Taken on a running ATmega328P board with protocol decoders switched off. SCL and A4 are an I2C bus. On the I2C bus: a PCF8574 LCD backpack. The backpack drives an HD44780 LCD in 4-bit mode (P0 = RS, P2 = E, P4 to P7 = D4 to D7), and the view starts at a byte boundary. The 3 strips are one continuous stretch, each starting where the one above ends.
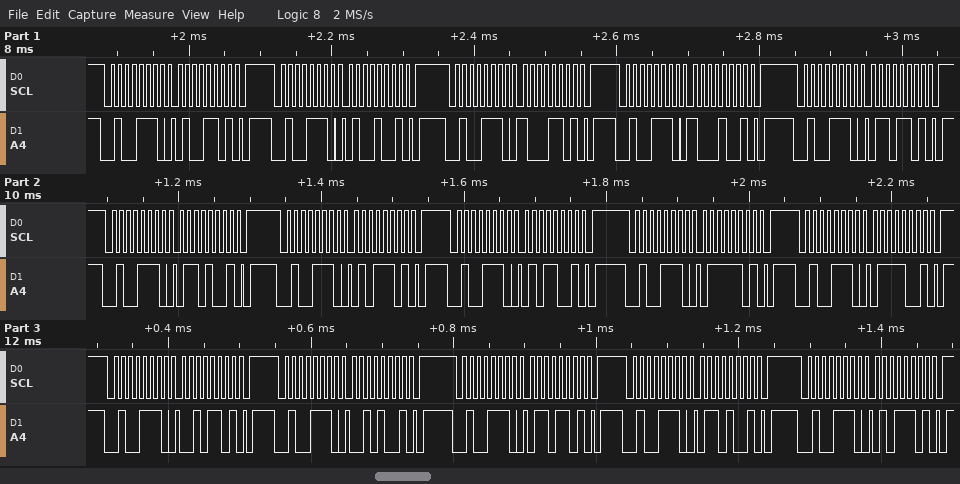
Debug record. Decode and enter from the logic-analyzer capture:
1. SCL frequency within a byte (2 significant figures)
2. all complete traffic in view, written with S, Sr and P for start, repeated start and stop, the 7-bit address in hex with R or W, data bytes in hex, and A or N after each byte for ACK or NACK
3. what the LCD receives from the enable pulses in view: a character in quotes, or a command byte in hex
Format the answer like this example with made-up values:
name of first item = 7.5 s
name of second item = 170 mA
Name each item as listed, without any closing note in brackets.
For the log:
SCL frequency within a byte = 100 kHz
all complete traffic in view, written with S, Sr and P for start, repeated start and stop, the 7-bit address in hex with R or W, data bytes in hex, and A or N after each byte for ACK or NACK = S 27W A 4D A P S 27W A 49 A P S 27W A 8D A P S 27W A 89 A P S 27W A 6D A P S 27W A 69 A P S 27W A 5D A P S 27W A 59 A P S 27W A 7D A P S 27W A 79 A P S 27W A 2D A P S 27W A 29 A P S 27W A 6D A P S 27W A 69 A P S 27W A 5D A P
what the LCD receives from the enable pulses in view: a character in quotes, or a command byte in hex = 'H' 'e' 'r'
